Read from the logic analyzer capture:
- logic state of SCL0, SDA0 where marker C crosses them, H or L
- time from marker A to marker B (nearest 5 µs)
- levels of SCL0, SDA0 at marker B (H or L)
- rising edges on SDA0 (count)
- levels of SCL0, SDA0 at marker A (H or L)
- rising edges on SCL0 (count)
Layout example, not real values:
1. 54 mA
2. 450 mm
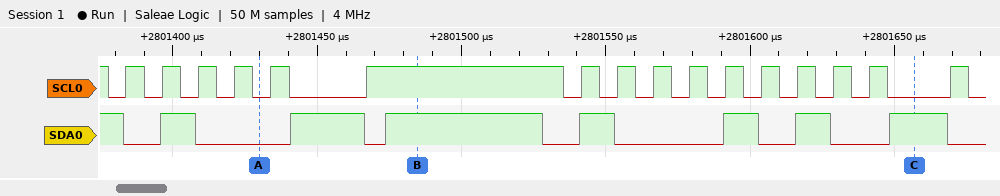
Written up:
1. SCL0=L, SDA0=H
2. 55 µs
3. SCL0=H, SDA0=H
4. 7
5. SCL0=L, SDA0=L
6. 16
